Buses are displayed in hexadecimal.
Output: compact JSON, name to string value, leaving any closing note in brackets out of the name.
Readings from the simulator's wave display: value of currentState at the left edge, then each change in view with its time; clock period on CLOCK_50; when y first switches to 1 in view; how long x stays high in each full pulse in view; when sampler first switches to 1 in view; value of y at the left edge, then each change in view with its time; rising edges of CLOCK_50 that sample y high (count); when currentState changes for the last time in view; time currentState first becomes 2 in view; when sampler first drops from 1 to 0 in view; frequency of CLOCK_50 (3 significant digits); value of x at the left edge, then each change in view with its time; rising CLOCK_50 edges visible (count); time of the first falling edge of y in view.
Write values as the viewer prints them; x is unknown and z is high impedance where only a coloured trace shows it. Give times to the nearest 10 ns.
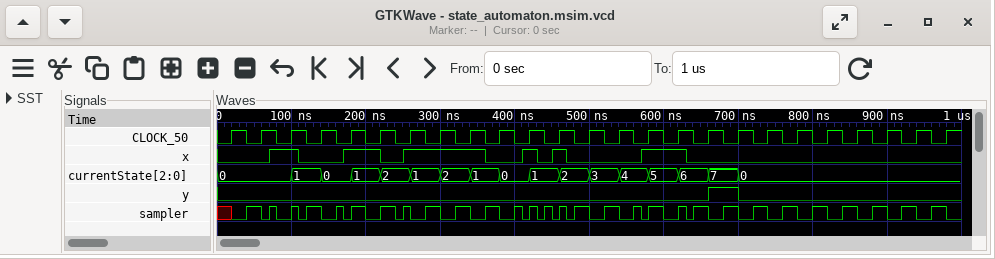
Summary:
{"value of currentState at the left edge, then each change in view with its time": "0, 1 at 100 ns, 0 at 140 ns, 1 at 180 ns, 2 at 220 ns, 1 at 260 ns, 2 at 300 ns, 1 at 340 ns, 0 at 380 ns, 1 at 420 ns, 2 at 460 ns, 3 at 500 ns, 4 at 540 ns, 5 at 580 ns, 6 at 620 ns, 7 at 660 ns, 0 at 700 ns", "clock period on CLOCK_50": "40 ns", "when y first switches to 1 in view": "660 ns", "how long x stays high in each full pulse in view": "40 ns, 50 ns, 110 ns, 20 ns, 20 ns, 60 ns", "when sampler first switches to 1 in view": "40 ns", "value of y at the left edge, then each change in view with its time": "0, 1 at 660 ns, 0 at 700 ns", "rising edges of CLOCK_50 that sample y high": "1", "when currentState changes for the last time in view": "700 ns", "time currentState first becomes 2 in view": "220 ns", "when sampler first drops from 1 to 0 in view": "60 ns", "frequency of CLOCK_50": "25.0 MHz", "value of x at the left edge, then each change in view with its time": "0, 1 at 70 ns, 0 at 110 ns, 1 at 170 ns, 0 at 220 ns, 1 at 250 ns, 0 at 360 ns, 1 at 410 ns, 0 at 430 ns, 1 at 450 ns, 0 at 470 ns, 1 at 570 ns, 0 at 630 ns", "rising CLOCK_50 edges visible": "25", "time of the first falling edge of y in view": "700 ns"}
